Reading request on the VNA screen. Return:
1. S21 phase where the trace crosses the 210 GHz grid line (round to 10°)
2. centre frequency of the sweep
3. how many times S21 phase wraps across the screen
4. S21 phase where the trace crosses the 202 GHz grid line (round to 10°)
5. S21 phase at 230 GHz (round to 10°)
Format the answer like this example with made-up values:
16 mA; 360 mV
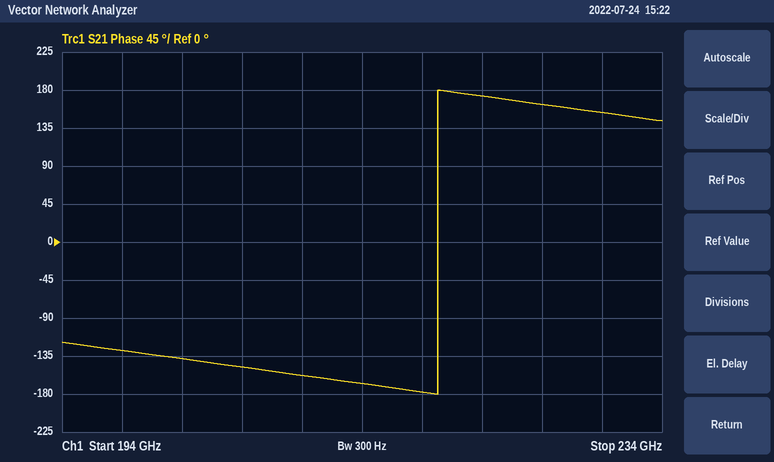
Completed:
-160°; 214 GHz; 1; -140°; 150°
